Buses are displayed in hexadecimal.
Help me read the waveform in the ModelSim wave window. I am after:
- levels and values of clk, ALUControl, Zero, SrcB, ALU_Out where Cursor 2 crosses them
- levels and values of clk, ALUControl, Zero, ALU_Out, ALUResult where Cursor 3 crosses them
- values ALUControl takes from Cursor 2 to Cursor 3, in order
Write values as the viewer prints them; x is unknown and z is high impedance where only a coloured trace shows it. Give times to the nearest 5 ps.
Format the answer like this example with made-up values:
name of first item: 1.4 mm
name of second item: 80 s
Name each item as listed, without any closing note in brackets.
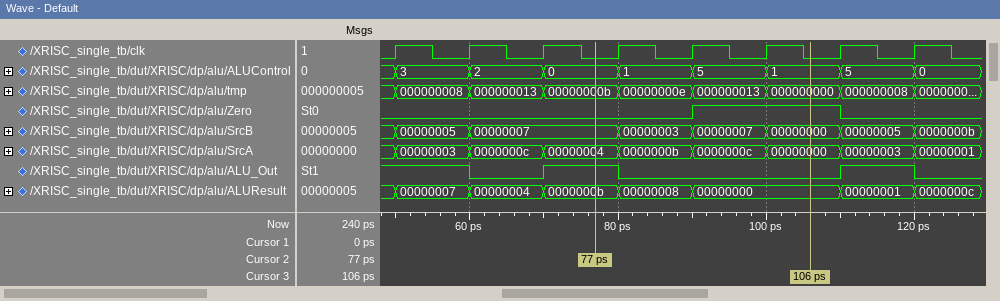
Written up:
levels and values of clk, ALUControl, Zero, SrcB, ALU_Out where Cursor 2 crosses them: clk=0, ALUControl=0, Zero=0, SrcB=00000007, ALU_Out=1
levels and values of clk, ALUControl, Zero, ALU_Out, ALUResult where Cursor 3 crosses them: clk=0, ALUControl=1, Zero=1, ALU_Out=0, ALUResult=00000000
values ALUControl takes from Cursor 2 to Cursor 3, in order: 0, 1, 5, 1
